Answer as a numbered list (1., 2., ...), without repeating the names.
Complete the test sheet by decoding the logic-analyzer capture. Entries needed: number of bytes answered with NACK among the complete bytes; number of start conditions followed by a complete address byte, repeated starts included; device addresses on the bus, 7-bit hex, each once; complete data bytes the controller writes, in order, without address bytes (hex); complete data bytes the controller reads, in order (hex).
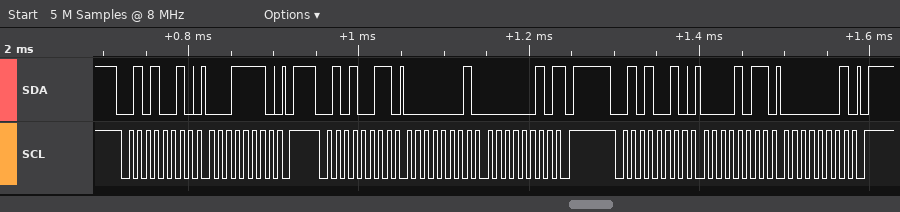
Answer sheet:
1. 1
2. 3
3. 0x29
4. 1E 0B 01
5. 01 02
